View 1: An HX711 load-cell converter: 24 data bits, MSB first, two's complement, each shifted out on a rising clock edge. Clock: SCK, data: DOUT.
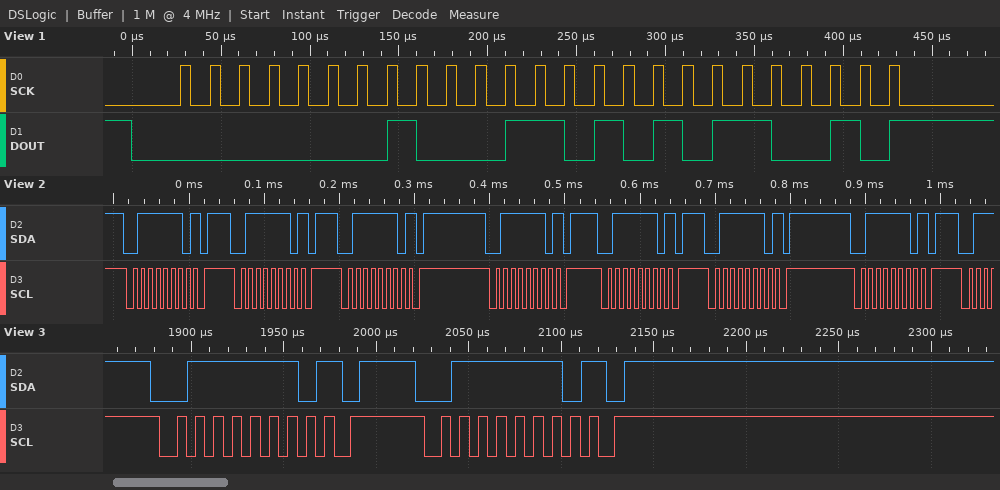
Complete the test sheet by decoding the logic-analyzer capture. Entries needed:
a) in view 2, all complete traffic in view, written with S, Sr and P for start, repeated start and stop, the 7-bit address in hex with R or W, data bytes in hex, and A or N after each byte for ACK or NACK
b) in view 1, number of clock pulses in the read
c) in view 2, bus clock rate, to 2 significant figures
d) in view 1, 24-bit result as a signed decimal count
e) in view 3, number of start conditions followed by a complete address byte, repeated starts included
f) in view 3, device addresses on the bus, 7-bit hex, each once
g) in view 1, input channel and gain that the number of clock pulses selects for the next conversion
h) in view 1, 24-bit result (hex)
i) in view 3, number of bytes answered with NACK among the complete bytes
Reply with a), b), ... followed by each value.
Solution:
a) S 3FW N P S 3FW N P S 3FW N P S 3FW N P S 3FW N P S 3FW N P S 3FW N P
b) 25
c) 100 kHz
d) 72370
e) 2
f) 0x3F
g) channel A, gain 128
h) 0x011AB2
i) 2
